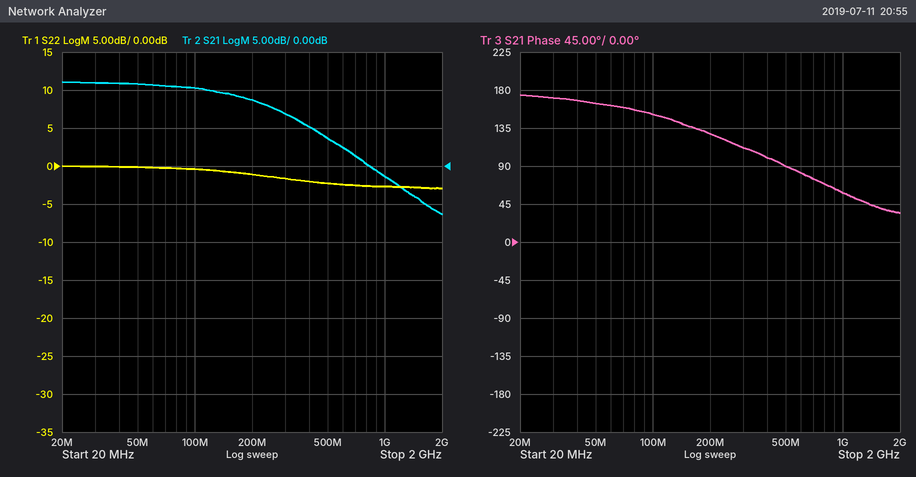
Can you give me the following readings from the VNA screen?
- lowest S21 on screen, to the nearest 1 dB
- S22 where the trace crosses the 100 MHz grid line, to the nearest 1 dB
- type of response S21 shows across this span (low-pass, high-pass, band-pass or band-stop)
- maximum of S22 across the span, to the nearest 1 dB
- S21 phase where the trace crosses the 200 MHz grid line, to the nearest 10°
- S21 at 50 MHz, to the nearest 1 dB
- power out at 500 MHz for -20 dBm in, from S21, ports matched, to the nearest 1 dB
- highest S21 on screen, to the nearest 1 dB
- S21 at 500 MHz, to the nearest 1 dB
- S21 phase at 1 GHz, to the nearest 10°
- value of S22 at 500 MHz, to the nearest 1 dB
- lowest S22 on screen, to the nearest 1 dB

-6 dB
0 dB
low-pass
0 dB
130°
11 dB
-16 dBm
11 dB
4 dB
60°
-2 dB
-3 dB
